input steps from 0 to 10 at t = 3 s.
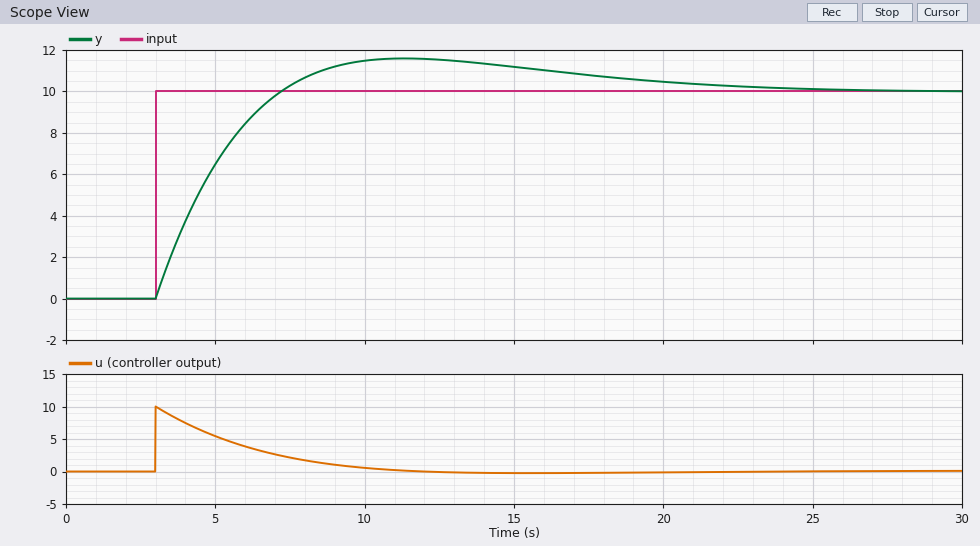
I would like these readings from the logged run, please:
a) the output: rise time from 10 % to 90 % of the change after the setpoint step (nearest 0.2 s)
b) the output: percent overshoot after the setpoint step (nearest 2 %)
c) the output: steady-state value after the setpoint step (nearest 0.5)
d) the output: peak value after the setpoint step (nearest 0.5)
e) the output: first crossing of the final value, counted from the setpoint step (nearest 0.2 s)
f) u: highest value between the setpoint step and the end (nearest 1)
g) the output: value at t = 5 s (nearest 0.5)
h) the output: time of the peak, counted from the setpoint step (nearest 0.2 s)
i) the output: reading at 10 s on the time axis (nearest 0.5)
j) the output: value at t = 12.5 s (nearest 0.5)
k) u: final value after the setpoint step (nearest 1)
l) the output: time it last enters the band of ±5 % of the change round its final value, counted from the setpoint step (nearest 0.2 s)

3.2 s
16 %
10.0
11.5
4.2 s
10
6.5
8.4 s
11.5
11.5
0
16.6 s
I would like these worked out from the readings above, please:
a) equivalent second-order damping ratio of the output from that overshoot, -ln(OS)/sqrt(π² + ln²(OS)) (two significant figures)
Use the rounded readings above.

0.50
